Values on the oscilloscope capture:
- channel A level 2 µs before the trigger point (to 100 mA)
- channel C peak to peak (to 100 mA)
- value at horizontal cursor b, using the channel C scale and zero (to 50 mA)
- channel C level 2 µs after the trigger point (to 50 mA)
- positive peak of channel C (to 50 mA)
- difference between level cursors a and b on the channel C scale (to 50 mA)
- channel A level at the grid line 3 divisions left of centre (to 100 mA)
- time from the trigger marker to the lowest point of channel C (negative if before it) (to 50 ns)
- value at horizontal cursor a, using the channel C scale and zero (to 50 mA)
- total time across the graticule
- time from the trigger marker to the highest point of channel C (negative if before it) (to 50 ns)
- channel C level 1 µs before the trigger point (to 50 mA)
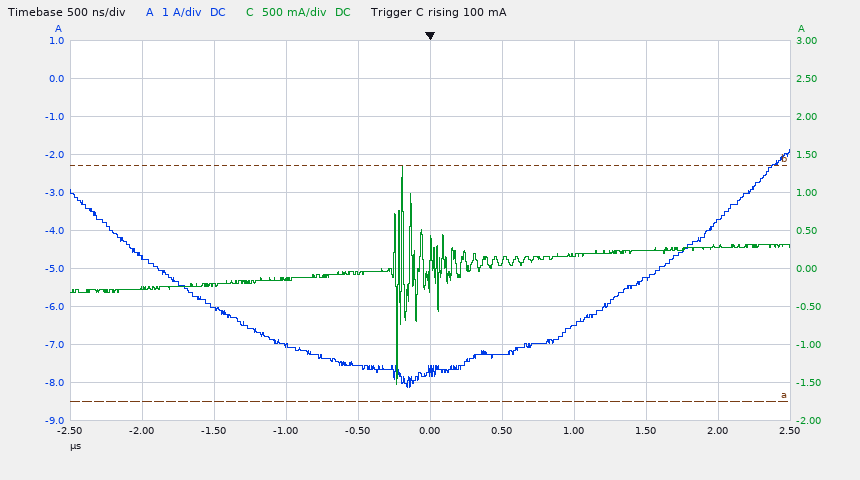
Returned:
-4.7 A
2.90 A
1.35 A
300 mA
1.35 A
3.10 A
-6.1 A
-250 ns
-1.75 A
5 µs
-200 ns
-150 mA
